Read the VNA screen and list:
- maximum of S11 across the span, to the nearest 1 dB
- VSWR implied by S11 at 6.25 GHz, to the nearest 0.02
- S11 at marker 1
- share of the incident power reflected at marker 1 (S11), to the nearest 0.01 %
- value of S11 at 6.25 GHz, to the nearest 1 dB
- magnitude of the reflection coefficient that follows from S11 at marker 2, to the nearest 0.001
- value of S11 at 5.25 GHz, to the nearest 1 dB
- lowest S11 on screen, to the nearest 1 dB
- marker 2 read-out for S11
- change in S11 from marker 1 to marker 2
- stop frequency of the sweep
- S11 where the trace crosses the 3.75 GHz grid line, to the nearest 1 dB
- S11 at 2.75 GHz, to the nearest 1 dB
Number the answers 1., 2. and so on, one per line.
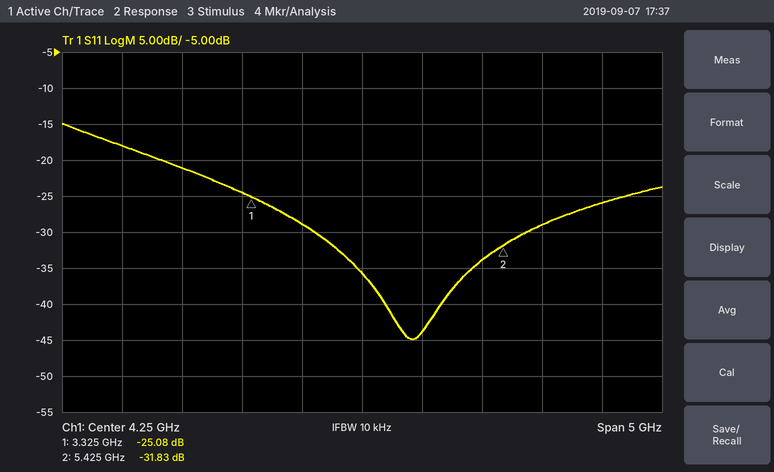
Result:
1. -15 dB
2. 1.10
3. -25.08 dB
4. 0.31 %
5. -26 dB
6. 0.026
7. -34 dB
8. -45 dB
9. -31.83 dB
10. -6.75 dB
11. 6.75 GHz
12. -29 dB
13. -21 dB
